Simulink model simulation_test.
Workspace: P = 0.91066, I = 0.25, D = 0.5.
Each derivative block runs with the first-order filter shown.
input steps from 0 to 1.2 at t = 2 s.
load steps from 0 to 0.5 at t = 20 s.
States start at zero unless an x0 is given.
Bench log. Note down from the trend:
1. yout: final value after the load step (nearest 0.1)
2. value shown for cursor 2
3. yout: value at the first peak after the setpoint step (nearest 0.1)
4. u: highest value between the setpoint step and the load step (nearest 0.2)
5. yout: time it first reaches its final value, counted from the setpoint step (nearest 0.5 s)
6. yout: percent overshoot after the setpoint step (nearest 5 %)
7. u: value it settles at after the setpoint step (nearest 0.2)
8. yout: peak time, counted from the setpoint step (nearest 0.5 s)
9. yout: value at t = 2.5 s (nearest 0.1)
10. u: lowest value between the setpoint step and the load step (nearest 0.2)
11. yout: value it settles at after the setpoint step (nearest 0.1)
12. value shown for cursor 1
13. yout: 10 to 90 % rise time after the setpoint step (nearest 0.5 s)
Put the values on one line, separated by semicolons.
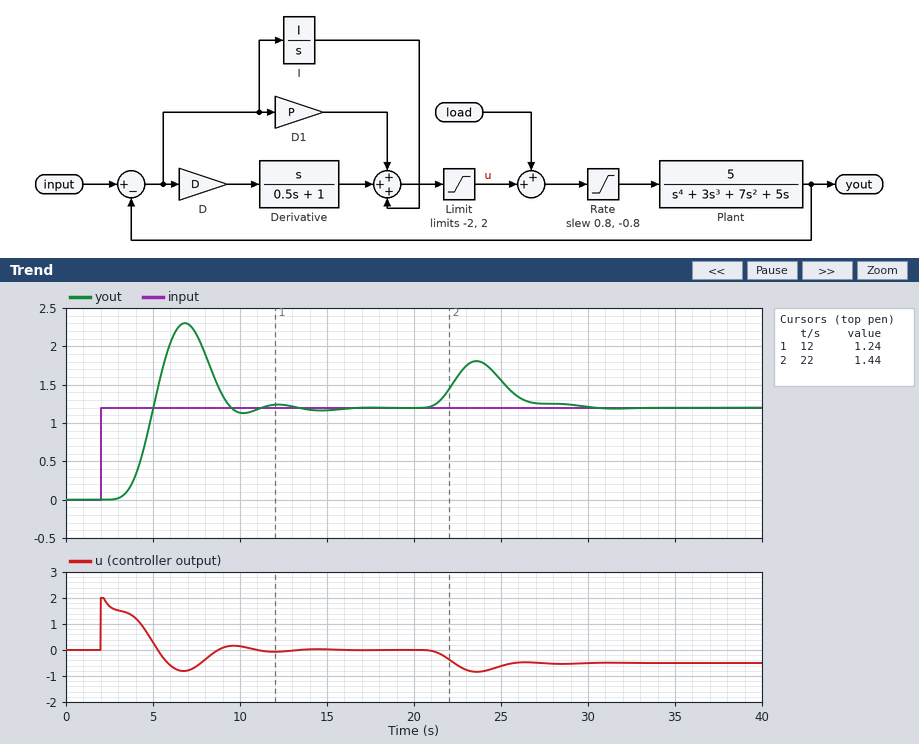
1.2; 1.44; 2.3; 2.0; 3.0 s; 90 %; 0.0; 5.0 s; 0.0; -0.8; 1.2; 1.24; 1.5 s
